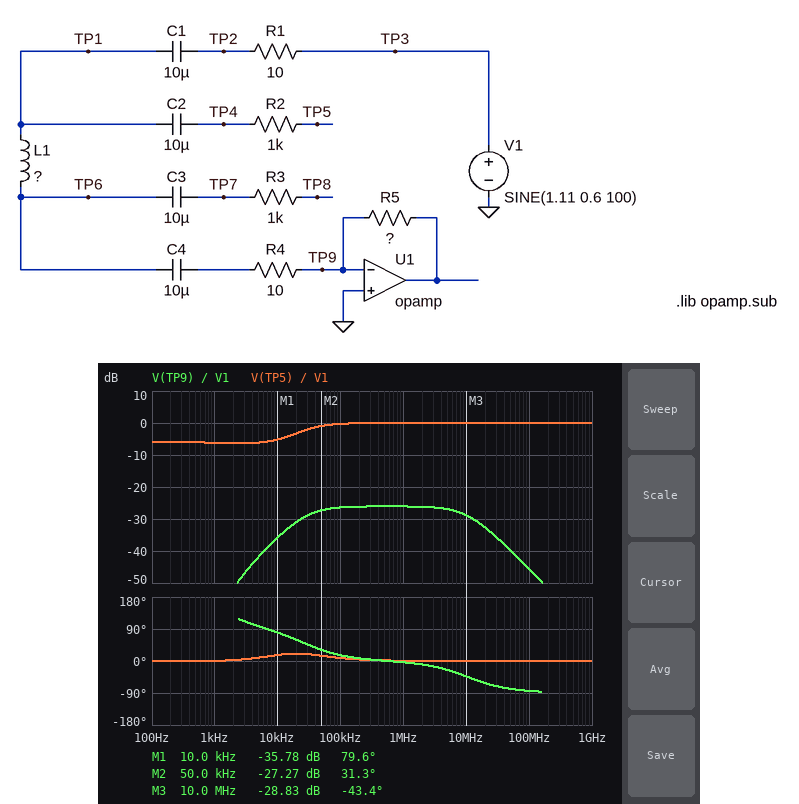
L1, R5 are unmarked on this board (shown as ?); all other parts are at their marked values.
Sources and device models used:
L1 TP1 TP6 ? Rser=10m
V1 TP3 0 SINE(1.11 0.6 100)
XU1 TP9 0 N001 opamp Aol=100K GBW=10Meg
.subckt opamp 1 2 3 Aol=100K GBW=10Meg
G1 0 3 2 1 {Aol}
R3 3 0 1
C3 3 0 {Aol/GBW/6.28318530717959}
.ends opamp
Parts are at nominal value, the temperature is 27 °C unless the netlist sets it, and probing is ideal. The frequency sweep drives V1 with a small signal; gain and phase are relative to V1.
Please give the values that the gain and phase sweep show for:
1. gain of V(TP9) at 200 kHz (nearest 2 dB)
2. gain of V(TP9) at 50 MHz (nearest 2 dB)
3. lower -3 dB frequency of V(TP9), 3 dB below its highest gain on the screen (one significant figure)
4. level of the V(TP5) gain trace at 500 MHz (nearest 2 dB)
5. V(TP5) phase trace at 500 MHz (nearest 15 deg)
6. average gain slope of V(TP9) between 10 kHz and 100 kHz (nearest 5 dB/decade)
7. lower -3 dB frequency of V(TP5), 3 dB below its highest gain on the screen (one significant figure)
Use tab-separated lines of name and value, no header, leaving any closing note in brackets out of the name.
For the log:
gain of V(TP9) at 200 kHz	-26 dB
gain of V(TP9) at 50 MHz	-40 dB
lower -3 dB frequency of V(TP9), 3 dB below its highest gain on the screen	30 kHz
level of the V(TP5) gain trace at 500 MHz	0 dB
V(TP5) phase trace at 500 MHz	0 deg
average gain slope of V(TP9) between 10 kHz and 100 kHz	10 dB/decade
lower -3 dB frequency of V(TP5), 3 dB below its highest gain on the screen	20 kHz
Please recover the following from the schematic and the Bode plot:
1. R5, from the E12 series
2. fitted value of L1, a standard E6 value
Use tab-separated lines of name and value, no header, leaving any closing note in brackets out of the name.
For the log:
R5, from the E12 series	330 Ω
fitted value of L1, a standard E6 value	100 µH
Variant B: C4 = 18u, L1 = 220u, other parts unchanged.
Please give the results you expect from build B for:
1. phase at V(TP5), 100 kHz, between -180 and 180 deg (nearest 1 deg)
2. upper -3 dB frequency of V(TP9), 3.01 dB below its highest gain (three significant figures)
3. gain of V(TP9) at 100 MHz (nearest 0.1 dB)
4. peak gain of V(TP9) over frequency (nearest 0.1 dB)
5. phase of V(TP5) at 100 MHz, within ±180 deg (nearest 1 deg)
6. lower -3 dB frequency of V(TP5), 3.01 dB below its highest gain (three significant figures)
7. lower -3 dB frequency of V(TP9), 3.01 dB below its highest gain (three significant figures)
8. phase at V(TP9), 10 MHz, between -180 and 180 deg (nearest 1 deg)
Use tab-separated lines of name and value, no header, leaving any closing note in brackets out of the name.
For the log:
phase at V(TP5), 100 kHz, between -180 and 180 deg	4 deg
upper -3 dB frequency of V(TP9), 3.01 dB below its highest gain	10.3 MHz
gain of V(TP9) at 100 MHz	-52.5 dB
peak gain of V(TP9) over frequency	-32.7 dB
phase of V(TP5) at 100 MHz, within ±180 deg	0 deg
lower -3 dB frequency of V(TP5), 3.01 dB below its highest gain	9.61 kHz
lower -3 dB frequency of V(TP9), 3.01 dB below its highest gain	12.9 kHz
phase at V(TP9), 10 MHz, between -180 and 180 deg	-44 deg
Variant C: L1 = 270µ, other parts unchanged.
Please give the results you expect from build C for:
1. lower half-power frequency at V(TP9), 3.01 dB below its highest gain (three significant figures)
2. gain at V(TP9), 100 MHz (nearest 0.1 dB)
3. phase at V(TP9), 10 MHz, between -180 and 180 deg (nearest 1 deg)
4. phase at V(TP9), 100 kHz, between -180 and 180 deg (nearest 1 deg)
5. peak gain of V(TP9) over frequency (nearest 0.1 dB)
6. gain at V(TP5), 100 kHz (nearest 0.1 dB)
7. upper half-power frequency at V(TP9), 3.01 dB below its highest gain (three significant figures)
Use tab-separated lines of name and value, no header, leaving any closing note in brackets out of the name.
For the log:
lower half-power frequency at V(TP9), 3.01 dB below its highest gain	10.0 kHz
gain at V(TP9), 100 MHz	-54.3 dB
phase at V(TP9), 10 MHz, between -180 and 180 deg	-44 deg
phase at V(TP9), 100 kHz, between -180 and 180 deg	6 deg
peak gain of V(TP9) over frequency	-34.4 dB
gain at V(TP5), 100 kHz	0 dB
upper half-power frequency at V(TP9), 3.01 dB below its highest gain	10.2 MHz
